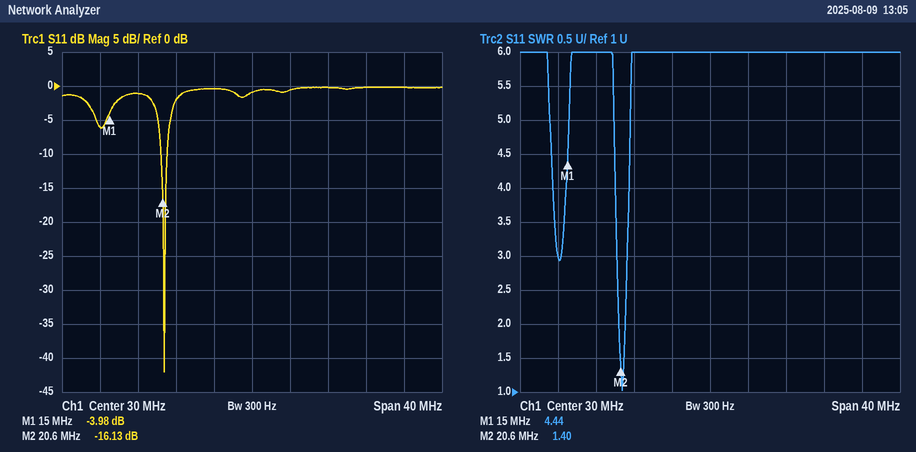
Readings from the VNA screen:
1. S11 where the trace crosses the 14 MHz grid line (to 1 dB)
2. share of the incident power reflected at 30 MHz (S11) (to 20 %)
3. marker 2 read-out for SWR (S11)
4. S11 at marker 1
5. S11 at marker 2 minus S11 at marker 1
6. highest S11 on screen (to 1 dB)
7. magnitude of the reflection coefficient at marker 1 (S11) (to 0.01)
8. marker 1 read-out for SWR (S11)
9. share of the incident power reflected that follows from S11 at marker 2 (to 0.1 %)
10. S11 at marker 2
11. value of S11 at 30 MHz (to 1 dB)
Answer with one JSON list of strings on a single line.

["-6 dB", "80 %", "1.40", "-3.98 dB", "-12.15 dB", "0 dB", "0.63", "4.44", "2.4 %", "-16.13 dB", "-1 dB"]
